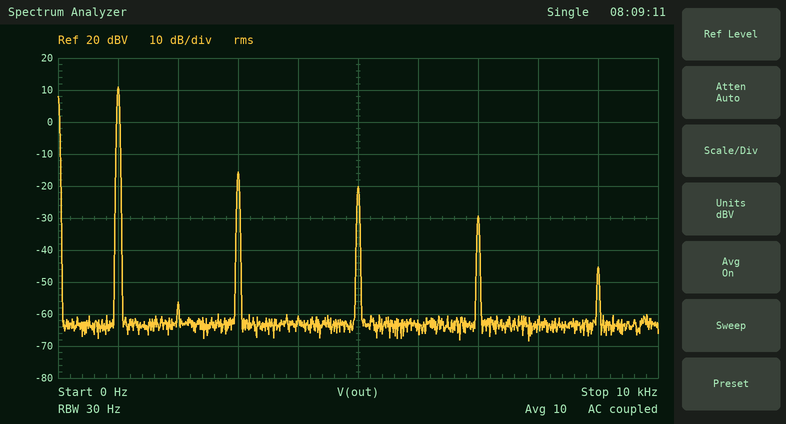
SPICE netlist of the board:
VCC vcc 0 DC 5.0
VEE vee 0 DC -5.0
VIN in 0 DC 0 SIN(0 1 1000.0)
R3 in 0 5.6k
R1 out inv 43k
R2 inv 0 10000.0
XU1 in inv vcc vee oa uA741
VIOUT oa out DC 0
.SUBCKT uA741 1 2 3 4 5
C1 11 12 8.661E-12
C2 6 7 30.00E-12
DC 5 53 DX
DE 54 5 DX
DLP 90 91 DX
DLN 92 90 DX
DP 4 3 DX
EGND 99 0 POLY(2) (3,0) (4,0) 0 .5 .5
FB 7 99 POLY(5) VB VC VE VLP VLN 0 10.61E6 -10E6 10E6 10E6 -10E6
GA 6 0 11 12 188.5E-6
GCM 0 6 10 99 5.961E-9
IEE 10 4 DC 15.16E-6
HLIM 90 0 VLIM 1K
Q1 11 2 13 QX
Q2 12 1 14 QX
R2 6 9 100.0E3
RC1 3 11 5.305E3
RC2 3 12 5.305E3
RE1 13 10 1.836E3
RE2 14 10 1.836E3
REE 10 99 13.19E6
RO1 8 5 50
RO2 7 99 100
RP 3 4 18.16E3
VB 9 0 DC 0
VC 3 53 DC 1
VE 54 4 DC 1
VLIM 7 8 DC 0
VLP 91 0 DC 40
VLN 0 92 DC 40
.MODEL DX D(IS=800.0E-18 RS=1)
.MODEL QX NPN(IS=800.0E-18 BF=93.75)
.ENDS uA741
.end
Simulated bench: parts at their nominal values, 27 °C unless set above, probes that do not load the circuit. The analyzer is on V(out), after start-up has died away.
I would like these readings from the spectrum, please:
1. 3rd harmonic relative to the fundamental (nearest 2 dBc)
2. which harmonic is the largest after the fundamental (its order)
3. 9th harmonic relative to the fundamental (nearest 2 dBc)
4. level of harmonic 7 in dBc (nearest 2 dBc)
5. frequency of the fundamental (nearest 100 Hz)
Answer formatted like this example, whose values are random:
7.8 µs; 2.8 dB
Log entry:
-26 dBc; 3; -56 dBc; -40 dBc; 1.0 kHz
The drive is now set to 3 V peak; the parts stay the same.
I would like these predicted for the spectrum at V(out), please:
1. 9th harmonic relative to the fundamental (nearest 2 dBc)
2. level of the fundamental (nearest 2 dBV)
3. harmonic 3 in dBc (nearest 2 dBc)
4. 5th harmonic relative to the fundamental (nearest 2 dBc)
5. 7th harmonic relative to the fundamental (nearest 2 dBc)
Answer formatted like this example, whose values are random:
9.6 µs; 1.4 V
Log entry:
-34 dBc; 12 dBV; -10 dBc; -18 dBc; -24 dBc
